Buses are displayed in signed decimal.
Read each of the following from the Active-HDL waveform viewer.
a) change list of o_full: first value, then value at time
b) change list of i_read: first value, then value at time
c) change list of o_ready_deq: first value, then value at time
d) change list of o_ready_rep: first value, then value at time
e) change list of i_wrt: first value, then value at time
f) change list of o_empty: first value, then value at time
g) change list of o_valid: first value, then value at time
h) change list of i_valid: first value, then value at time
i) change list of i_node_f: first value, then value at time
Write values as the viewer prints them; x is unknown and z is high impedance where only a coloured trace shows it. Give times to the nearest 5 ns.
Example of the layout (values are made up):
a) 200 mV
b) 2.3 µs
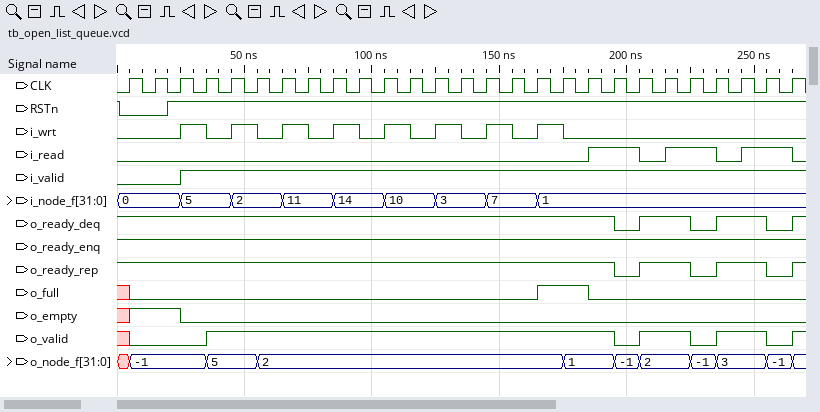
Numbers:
a) x, 0 at 5 ns, 1 at 165 ns, 0 at 185 ns
b) 0, 1 at 185 ns, 0 at 205 ns, 1 at 215 ns, 0 at 235 ns, 1 at 245 ns, 0 at 265 ns
c) 1, 0 at 195 ns, 1 at 205 ns, 0 at 225 ns, 1 at 235 ns, 0 at 255 ns, 1 at 265 ns
d) 1, 0 at 195 ns, 1 at 205 ns, 0 at 225 ns, 1 at 235 ns, 0 at 255 ns, 1 at 265 ns
e) 0, 1 at 25 ns, 0 at 35 ns, 1 at 45 ns, 0 at 55 ns, 1 at 65 ns, 0 at 75 ns, 1 at 85 ns, 0 at 95 ns, 1 at 105 ns, 0 at 115 ns, 1 at 125 ns, 0 at 135 ns, 1 at 145 ns, 0 at 155 ns, 1 at 165 ns, 0 at 175 ns
f) x, 1 at 5 ns, 0 at 25 ns
g) x, 0 at 5 ns, 1 at 35 ns, 0 at 195 ns, 1 at 205 ns, 0 at 225 ns, 1 at 235 ns, 0 at 255 ns, 1 at 265 ns
h) 0, 1 at 25 ns
i) 0, 5 at 25 ns, 2 at 45 ns, 11 at 65 ns, 14 at 85 ns, 10 at 105 ns, 3 at 125 ns, 7 at 145 ns, 1 at 165 ns
